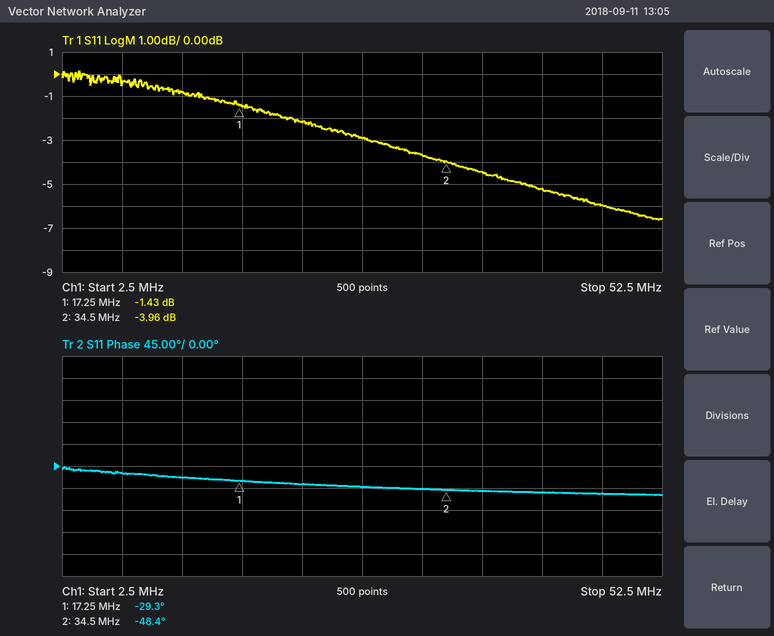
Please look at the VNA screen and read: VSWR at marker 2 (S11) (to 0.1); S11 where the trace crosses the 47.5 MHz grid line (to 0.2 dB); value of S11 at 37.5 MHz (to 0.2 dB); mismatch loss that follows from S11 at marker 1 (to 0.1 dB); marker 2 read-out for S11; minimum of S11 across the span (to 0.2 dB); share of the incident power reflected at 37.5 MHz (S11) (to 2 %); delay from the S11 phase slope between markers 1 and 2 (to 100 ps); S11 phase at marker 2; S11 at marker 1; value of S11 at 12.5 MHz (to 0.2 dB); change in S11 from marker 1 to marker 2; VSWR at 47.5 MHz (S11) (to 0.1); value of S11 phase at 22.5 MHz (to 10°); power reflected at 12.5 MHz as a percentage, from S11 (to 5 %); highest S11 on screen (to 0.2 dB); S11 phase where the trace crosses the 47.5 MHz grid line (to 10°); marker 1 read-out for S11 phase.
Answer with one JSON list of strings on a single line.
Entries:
["4.5", "-6.0 dB", "-4.4 dB", "5.5 dB", "-3.96 dB", "-6.6 dB", "36 %", "3.1 ns", "-48.4°", "-1.43 dB", "-0.8 dB", "-2.53 dB", "3.0", "-40°", "85 %", "0.2 dB", "-60°", "-29.3°"]
